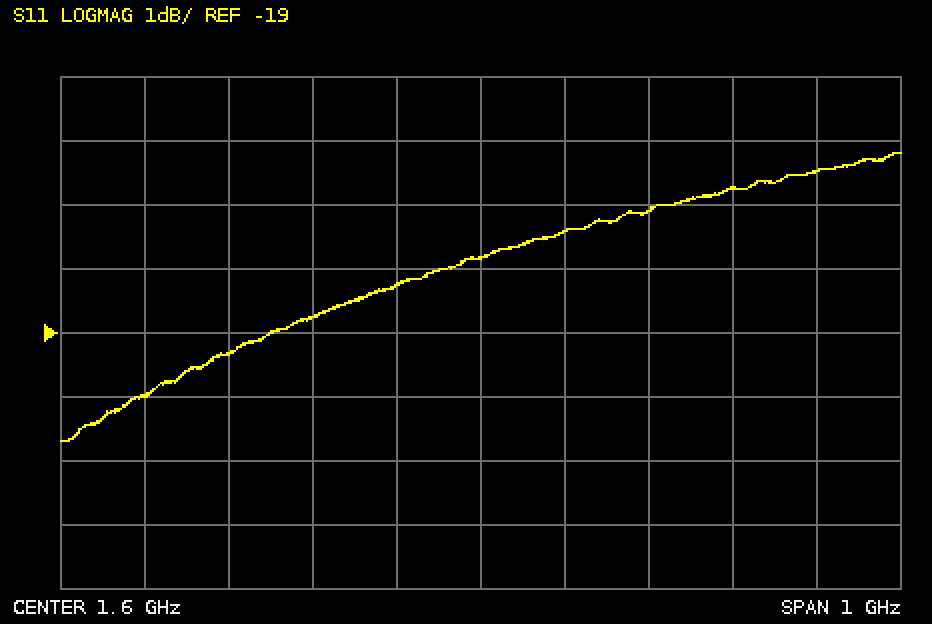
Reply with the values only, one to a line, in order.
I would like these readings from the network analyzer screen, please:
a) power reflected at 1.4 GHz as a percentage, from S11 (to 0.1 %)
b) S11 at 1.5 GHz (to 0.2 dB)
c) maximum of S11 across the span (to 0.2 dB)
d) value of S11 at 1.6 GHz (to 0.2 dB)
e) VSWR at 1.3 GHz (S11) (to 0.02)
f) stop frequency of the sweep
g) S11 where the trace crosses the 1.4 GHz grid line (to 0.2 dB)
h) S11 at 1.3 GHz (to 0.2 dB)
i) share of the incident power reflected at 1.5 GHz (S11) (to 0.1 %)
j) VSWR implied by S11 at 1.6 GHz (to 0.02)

1.3 %
-18.2 dB
-16.2 dB
-17.8 dB
1.24
2.1 GHz
-18.8 dB
-19.4 dB
1.5 %
1.30
